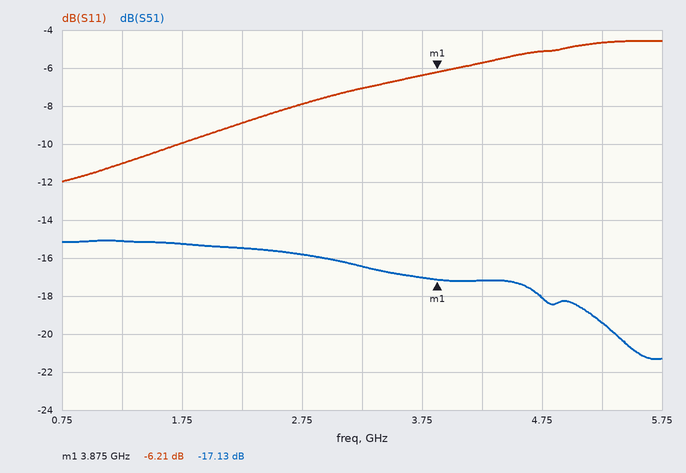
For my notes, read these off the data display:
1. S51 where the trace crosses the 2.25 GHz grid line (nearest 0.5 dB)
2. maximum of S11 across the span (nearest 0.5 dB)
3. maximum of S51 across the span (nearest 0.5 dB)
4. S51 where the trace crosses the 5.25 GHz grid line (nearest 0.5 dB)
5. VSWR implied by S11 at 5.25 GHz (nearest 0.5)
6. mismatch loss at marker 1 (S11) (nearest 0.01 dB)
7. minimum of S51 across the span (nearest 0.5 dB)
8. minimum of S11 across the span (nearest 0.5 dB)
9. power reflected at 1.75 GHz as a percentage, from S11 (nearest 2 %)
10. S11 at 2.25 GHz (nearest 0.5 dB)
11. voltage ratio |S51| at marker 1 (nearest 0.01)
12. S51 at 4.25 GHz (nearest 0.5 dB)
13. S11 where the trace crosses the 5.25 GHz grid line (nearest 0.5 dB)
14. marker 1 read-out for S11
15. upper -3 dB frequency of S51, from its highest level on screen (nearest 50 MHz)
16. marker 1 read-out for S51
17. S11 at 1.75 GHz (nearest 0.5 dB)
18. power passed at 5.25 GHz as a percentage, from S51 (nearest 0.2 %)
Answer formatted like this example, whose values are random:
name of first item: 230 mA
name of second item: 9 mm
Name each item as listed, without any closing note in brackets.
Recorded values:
S51 where the trace crosses the 2.25 GHz grid line: -15.5 dB
maximum of S11 across the span: -4.5 dB
maximum of S51 across the span: -15.0 dB
S51 where the trace crosses the 5.25 GHz grid line: -19.5 dB
VSWR implied by S11 at 5.25 GHz: 4.0
mismatch loss at marker 1 (S11): 1.19 dB
minimum of S51 across the span: -21.5 dB
minimum of S11 across the span: -12.0 dB
power reflected at 1.75 GHz as a percentage, from S11: 10 %
S11 at 2.25 GHz: -9.0 dB
voltage ratio |S51| at marker 1: 0.14
S51 at 4.25 GHz: -17.0 dB
S11 where the trace crosses the 5.25 GHz grid line: -4.5 dB
marker 1 read-out for S11: -6.21 dB
upper -3 dB frequency of S51, from its highest level on screen: 4.75 GHz
marker 1 read-out for S51: -17.13 dB
S11 at 1.75 GHz: -10.0 dB
power passed at 5.25 GHz as a percentage, from S51: 1.2 %
